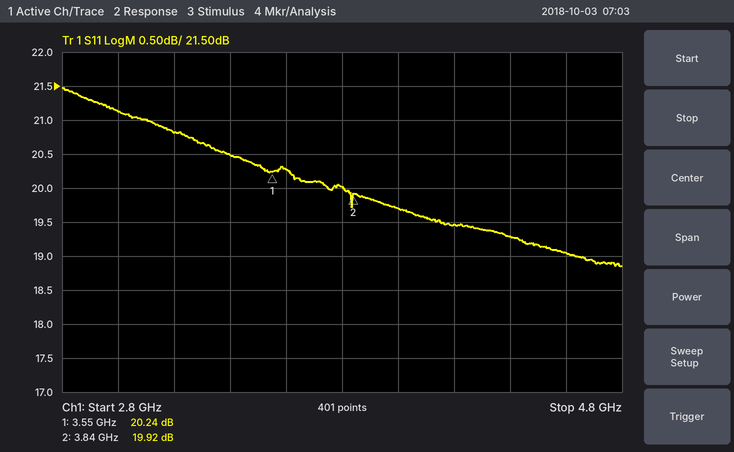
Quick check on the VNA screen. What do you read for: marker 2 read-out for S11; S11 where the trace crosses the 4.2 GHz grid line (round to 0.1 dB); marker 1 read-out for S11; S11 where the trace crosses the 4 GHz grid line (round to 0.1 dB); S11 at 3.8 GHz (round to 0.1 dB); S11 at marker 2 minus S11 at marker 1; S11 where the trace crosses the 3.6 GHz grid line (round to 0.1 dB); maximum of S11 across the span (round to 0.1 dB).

19.92 dB
19.5 dB
20.24 dB
19.7 dB
20.0 dB
-0.32 dB
20.3 dB
21.5 dB
